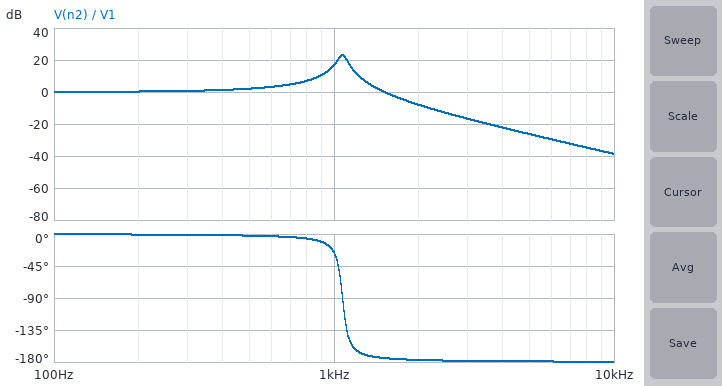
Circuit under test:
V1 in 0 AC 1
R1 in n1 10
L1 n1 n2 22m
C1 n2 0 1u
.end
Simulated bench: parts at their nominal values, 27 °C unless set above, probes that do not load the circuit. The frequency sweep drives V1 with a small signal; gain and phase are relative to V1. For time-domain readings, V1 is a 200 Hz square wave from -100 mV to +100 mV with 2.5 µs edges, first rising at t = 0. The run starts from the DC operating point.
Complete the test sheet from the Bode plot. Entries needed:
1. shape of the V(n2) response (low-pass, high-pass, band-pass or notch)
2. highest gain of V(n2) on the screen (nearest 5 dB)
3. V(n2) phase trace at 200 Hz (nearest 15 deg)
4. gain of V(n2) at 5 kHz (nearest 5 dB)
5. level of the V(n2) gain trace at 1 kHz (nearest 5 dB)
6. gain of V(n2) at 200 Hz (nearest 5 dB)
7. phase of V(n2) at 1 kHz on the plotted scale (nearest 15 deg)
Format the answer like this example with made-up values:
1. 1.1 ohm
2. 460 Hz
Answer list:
1. low-pass
2. 25 dB
3. 0 deg
4. -25 dB
5. 15 dB
6. 0 dB
7. -30 deg
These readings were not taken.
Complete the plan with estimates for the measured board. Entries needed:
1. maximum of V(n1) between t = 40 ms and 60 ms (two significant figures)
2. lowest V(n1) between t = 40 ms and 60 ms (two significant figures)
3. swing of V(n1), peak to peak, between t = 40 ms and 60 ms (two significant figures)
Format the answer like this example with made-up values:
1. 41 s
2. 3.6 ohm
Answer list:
1. 110 mV
2. -110 mV
3. 230 mV
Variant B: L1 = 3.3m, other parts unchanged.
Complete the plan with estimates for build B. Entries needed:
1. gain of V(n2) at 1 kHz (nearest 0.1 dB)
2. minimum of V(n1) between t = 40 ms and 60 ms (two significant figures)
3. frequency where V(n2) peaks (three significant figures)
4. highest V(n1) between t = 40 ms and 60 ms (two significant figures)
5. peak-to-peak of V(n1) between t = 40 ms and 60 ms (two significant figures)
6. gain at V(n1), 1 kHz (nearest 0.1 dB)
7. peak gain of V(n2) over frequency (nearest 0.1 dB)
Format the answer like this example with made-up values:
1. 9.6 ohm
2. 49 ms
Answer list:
1. 1.2 dB
2. -120 mV
3. 2.75 kHz
4. 120 mV
5. 250 mV
6. 0 dB
7. 15.2 dB
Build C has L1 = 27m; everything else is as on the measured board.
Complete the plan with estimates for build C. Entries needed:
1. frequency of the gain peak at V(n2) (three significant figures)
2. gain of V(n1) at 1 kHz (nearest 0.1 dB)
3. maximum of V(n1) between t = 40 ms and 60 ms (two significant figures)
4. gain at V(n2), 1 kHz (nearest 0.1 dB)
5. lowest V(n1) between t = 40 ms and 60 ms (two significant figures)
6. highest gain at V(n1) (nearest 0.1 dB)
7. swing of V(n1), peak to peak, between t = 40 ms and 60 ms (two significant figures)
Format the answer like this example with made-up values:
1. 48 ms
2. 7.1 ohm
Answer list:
1. 968 Hz
2. -2.8 dB
3. 120 mV
4. 20.8 dB
5. -120 mV
6. 0 dB
7. 240 mV
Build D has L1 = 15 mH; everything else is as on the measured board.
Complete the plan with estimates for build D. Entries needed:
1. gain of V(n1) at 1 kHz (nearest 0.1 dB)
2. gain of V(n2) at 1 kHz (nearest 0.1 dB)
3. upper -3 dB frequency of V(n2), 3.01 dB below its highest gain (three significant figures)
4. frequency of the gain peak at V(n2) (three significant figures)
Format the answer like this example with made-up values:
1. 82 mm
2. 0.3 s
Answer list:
1. -0.1 dB
2. 7.7 dB
3. 1.35 kHz
4. 1.30 kHz
